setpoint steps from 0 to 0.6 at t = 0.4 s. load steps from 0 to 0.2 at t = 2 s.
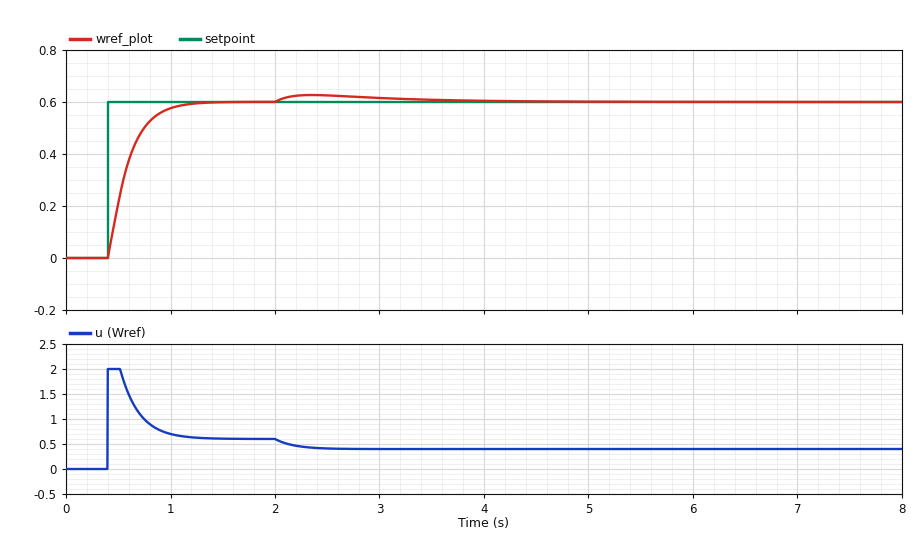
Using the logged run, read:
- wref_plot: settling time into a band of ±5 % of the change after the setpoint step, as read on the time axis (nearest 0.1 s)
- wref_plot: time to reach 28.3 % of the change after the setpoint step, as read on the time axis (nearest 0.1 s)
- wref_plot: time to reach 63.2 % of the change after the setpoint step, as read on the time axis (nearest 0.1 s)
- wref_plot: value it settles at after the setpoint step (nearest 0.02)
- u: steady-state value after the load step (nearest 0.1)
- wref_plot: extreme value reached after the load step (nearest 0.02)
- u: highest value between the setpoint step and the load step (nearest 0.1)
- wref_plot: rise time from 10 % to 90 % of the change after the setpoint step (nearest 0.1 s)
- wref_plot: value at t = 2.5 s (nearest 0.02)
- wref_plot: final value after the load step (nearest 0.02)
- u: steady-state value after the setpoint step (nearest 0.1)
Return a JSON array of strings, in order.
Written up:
["1.0 s", "0.5 s", "0.6 s", "0.60", "0.4", "0.62", "2.0", "0.4 s", "0.62", "0.60", "0.6"]
